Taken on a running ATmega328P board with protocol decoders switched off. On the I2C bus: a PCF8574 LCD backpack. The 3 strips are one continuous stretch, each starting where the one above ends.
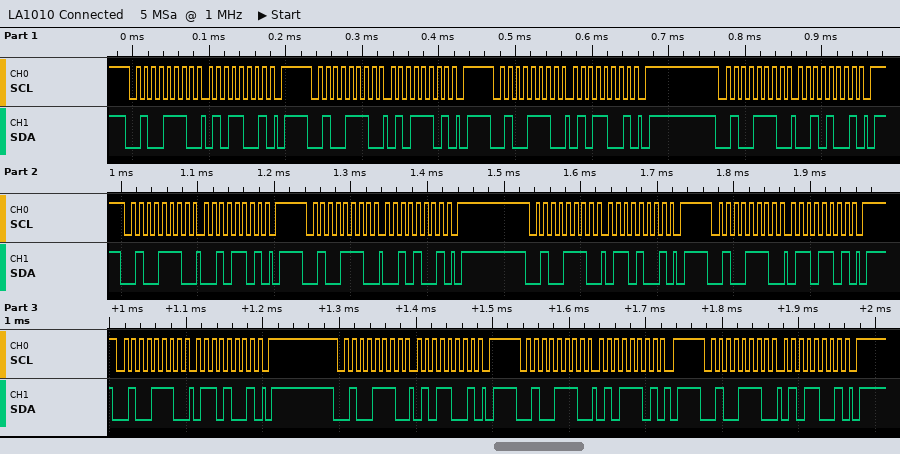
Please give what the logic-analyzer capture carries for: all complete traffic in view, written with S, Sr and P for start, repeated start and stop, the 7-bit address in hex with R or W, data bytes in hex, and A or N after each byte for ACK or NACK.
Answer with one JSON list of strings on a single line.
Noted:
["S 27W A 59 A P S 27W A 5D A P S 27W A 59 A P S 27W A 29 A P S 27W A 2D A P S 27W A 29 A P S 27W A 69 A P S 27W A 6D A P S 27W A 69 A P S 27W A 59 A P S 27W A 5D A P S 27W A 59 A P"]
